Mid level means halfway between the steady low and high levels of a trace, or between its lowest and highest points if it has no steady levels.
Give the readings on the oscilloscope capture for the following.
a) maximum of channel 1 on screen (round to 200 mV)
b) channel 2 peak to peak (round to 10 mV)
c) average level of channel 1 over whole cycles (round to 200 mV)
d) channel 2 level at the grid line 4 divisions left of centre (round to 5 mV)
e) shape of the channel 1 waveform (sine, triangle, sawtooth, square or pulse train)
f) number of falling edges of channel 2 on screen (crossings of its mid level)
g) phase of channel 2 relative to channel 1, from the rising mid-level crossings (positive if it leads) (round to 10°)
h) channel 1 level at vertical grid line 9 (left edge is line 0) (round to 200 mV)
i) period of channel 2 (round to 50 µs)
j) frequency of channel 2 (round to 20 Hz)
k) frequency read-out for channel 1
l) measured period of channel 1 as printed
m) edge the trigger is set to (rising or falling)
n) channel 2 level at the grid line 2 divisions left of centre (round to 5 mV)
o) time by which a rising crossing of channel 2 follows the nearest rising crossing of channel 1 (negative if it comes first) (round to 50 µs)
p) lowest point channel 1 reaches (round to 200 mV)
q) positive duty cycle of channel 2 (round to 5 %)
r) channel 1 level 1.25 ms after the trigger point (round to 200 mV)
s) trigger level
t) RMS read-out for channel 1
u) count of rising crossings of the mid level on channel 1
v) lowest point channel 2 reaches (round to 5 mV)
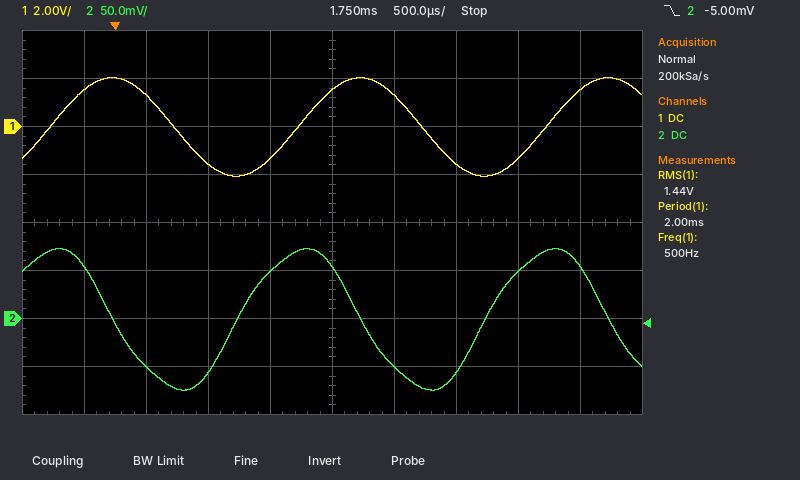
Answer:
2.0 V
150 mV
0.0 V
55 mV
sine
3
+90°
1.6 V
2.00 ms
500 Hz
500 Hz
2.00 ms
falling
-55 mV
-500 µs
-2.0 V
50 %
-1.4 V
-5.00 mV
1.44 V
3
-75 mV
